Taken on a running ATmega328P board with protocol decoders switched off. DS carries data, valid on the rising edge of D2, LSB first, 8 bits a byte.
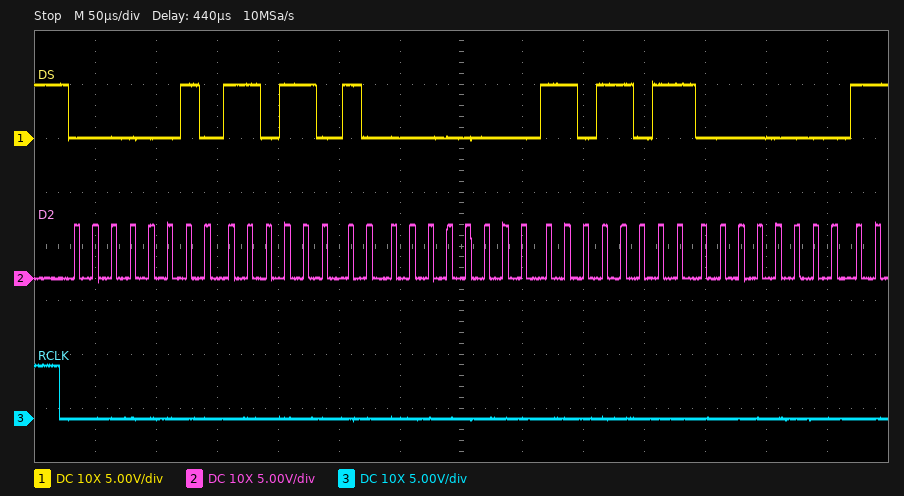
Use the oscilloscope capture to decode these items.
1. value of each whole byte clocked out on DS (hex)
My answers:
0x40 0x5B 0x00 0xDB 0x00
